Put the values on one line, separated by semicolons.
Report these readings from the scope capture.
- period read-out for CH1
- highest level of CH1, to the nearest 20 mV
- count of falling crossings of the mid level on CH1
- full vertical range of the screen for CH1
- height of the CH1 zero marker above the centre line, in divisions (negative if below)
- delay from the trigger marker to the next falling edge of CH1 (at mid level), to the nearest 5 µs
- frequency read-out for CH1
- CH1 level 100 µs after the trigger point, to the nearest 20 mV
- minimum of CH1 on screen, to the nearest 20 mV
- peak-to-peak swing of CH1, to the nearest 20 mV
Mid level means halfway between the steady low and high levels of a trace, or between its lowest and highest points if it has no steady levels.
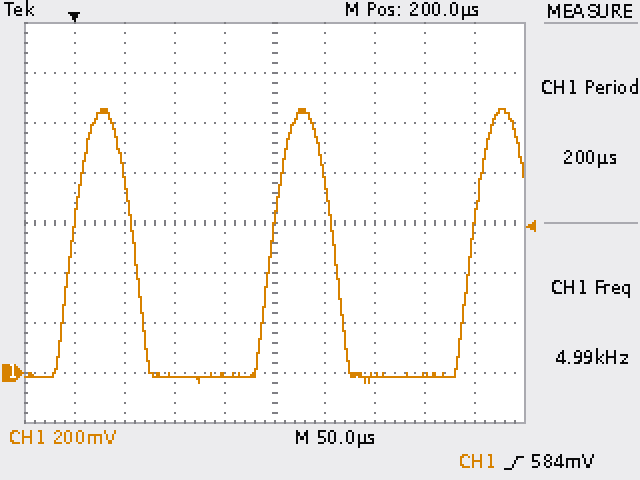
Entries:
200 µs; 1.06 V; 2; 1.6 V; -3.0 div; 60 µs; 4.99 kHz; -20 mV; -40 mV; 1.10 V
